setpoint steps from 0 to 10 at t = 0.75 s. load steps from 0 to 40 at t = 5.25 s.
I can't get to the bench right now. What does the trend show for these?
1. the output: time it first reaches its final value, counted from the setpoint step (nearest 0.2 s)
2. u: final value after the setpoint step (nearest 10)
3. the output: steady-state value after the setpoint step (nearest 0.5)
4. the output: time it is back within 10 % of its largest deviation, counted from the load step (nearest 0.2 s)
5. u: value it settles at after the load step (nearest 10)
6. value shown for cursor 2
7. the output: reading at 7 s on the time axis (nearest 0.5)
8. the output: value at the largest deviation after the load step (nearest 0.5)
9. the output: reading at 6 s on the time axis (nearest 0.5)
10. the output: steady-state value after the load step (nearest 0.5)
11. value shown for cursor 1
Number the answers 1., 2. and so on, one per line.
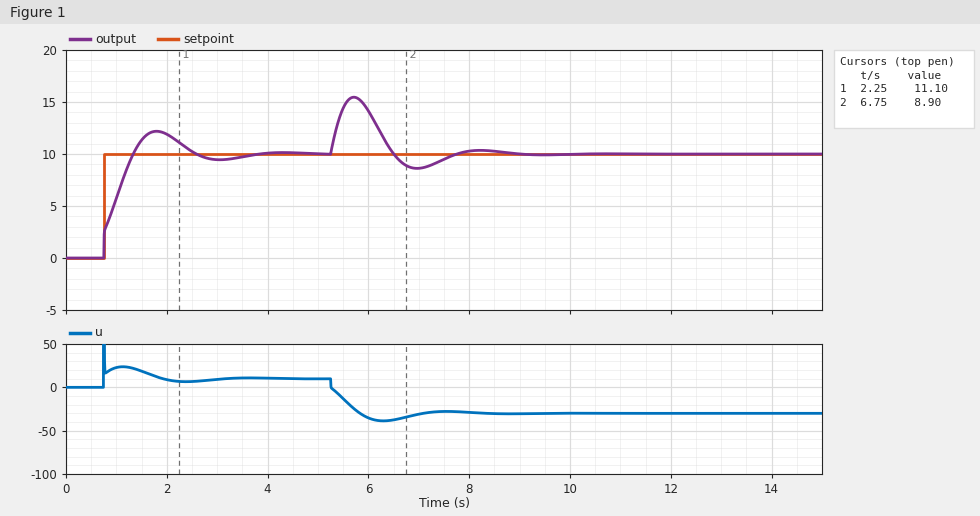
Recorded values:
1. 0.6 s
2. 10
3. 10.0
4. 2.2 s
5. -30
6. 8.90
7. 8.5
8. 15.5
9. 14.0
10. 10.0
11. 11.10
